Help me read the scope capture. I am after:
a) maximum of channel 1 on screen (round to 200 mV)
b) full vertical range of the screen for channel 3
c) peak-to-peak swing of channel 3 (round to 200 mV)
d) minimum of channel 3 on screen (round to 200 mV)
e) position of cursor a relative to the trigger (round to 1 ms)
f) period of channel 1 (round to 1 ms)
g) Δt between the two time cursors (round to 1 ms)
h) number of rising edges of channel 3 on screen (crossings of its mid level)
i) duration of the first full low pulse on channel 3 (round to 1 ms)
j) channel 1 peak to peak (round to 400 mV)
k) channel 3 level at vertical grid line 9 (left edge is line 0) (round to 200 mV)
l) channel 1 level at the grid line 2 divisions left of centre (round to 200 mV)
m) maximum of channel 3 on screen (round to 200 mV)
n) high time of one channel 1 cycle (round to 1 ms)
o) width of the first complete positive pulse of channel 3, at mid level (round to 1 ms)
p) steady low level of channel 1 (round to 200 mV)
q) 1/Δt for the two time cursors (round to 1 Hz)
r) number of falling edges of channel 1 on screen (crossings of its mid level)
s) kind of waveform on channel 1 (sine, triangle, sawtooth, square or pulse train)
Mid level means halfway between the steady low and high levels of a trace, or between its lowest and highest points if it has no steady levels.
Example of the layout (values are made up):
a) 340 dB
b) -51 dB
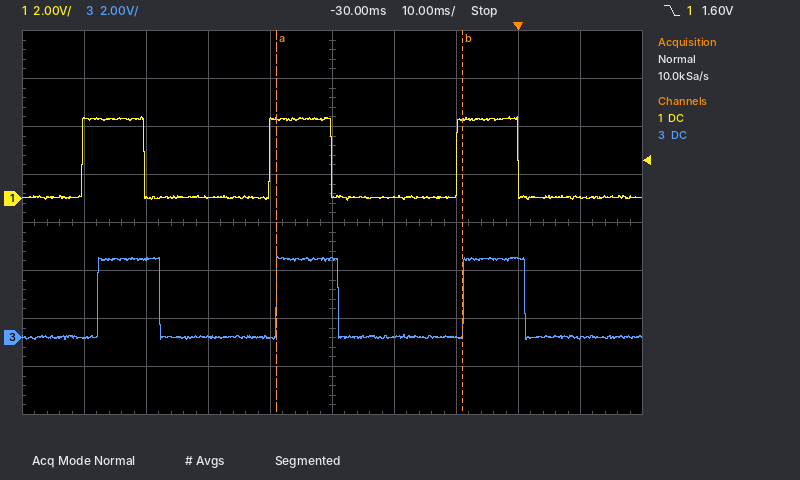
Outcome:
a) 3.4 V
b) 16 V
c) 3.4 V
d) 0.0 V
e) -39 ms
f) 30 ms
g) 30 ms
h) 3
i) 19 ms
j) 3.6 V
k) 0.0 V
l) 0.0 V
m) 3.4 V
n) 10 ms
o) 10 ms
p) 0.0 V
q) 33 Hz
r) 3
s) pulse train
